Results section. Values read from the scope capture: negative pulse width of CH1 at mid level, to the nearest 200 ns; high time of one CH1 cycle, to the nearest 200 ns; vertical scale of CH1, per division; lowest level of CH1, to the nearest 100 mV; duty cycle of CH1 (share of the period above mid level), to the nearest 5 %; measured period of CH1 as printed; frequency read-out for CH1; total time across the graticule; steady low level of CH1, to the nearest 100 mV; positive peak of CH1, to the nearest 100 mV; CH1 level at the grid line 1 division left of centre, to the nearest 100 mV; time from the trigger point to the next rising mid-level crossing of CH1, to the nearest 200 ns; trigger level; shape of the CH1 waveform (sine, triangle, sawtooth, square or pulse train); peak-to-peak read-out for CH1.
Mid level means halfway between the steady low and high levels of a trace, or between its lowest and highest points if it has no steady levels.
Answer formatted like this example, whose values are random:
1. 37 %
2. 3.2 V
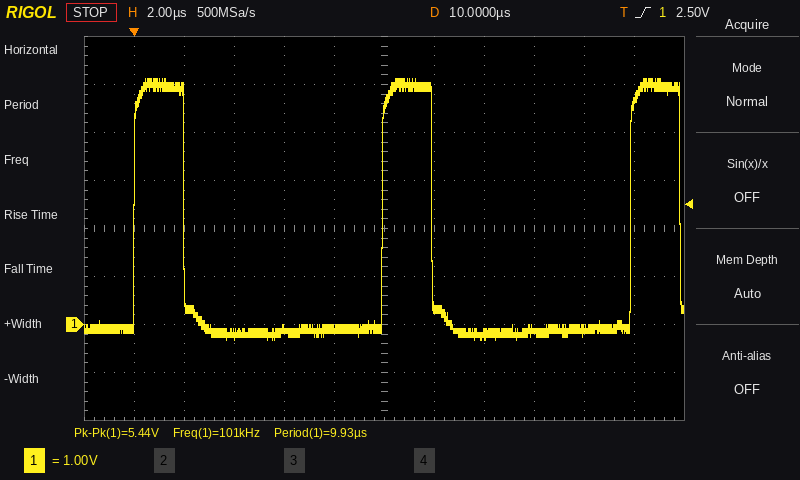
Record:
1. 8.0 µs
2. 2.0 µs
3. 1 V
4. -300 mV
5. 20 %
6. 9.93 µs
7. 101 kHz
8. 24 µs
9. -100 mV
10. 5.1 V
11. -100 mV
12. 10.0 µs
13. 2.50 V
14. pulse train
15. 5.44 V
